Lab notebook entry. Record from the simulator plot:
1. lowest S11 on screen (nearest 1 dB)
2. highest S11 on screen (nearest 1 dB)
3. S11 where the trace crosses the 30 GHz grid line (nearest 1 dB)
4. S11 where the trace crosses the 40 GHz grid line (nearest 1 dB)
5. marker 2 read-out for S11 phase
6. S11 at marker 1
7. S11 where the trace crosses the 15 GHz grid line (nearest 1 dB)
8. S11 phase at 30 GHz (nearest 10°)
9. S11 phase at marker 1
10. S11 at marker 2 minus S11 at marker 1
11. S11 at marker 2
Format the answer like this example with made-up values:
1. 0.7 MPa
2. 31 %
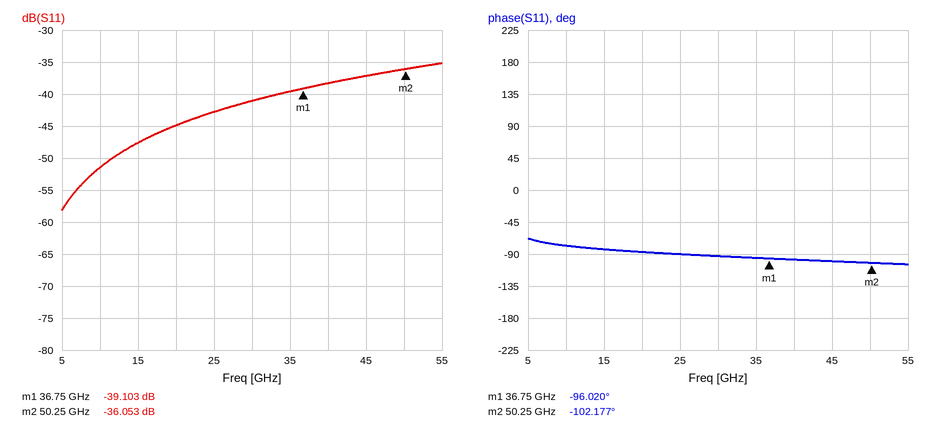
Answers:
1. -58 dB
2. -35 dB
3. -41 dB
4. -38 dB
5. -102.177°
6. -39.103 dB
7. -48 dB
8. -90°
9. -96.020°
10. 3.050 dB
11. -36.053 dB
